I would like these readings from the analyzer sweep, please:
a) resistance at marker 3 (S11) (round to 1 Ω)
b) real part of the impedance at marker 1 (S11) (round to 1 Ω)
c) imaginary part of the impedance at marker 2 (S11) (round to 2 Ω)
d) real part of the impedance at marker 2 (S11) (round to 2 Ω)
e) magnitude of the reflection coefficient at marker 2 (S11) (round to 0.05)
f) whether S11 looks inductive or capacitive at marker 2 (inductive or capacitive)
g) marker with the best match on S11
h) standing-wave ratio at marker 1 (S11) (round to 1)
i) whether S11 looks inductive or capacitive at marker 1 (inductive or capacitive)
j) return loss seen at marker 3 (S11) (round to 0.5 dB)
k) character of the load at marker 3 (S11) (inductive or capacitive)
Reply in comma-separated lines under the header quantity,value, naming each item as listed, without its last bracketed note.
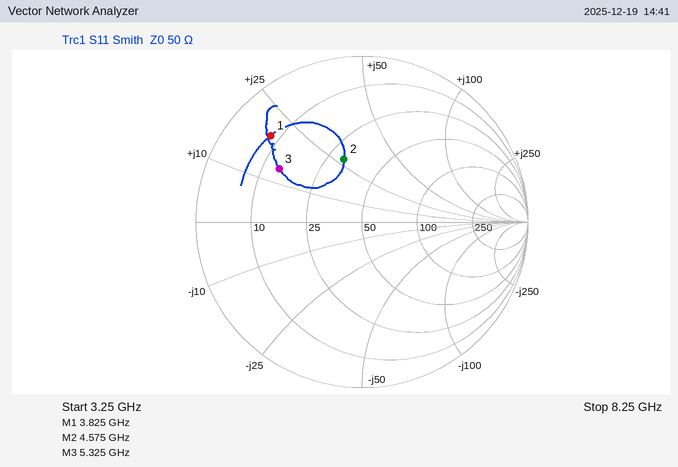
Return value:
quantity,value
resistance at marker 3 (S11),14 Ω
real part of the impedance at marker 1 (S11),8 Ω
imaginary part of the impedance at marker 2 (S11),+28 Ω
real part of the impedance at marker 2 (S11),30 Ω
magnitude of the reflection coefficient at marker 2 (S11),0.40
whether S11 looks inductive or capacitive at marker 2,inductive
marker with the best match on S11,marker 2
standing-wave ratio at marker 1 (S11),7
whether S11 looks inductive or capacitive at marker 1,inductive
return loss seen at marker 3 (S11),4.5 dB
character of the load at marker 3 (S11),inductive
